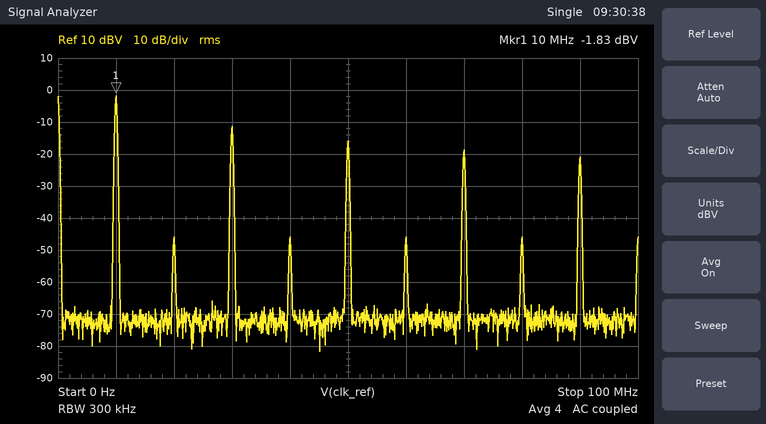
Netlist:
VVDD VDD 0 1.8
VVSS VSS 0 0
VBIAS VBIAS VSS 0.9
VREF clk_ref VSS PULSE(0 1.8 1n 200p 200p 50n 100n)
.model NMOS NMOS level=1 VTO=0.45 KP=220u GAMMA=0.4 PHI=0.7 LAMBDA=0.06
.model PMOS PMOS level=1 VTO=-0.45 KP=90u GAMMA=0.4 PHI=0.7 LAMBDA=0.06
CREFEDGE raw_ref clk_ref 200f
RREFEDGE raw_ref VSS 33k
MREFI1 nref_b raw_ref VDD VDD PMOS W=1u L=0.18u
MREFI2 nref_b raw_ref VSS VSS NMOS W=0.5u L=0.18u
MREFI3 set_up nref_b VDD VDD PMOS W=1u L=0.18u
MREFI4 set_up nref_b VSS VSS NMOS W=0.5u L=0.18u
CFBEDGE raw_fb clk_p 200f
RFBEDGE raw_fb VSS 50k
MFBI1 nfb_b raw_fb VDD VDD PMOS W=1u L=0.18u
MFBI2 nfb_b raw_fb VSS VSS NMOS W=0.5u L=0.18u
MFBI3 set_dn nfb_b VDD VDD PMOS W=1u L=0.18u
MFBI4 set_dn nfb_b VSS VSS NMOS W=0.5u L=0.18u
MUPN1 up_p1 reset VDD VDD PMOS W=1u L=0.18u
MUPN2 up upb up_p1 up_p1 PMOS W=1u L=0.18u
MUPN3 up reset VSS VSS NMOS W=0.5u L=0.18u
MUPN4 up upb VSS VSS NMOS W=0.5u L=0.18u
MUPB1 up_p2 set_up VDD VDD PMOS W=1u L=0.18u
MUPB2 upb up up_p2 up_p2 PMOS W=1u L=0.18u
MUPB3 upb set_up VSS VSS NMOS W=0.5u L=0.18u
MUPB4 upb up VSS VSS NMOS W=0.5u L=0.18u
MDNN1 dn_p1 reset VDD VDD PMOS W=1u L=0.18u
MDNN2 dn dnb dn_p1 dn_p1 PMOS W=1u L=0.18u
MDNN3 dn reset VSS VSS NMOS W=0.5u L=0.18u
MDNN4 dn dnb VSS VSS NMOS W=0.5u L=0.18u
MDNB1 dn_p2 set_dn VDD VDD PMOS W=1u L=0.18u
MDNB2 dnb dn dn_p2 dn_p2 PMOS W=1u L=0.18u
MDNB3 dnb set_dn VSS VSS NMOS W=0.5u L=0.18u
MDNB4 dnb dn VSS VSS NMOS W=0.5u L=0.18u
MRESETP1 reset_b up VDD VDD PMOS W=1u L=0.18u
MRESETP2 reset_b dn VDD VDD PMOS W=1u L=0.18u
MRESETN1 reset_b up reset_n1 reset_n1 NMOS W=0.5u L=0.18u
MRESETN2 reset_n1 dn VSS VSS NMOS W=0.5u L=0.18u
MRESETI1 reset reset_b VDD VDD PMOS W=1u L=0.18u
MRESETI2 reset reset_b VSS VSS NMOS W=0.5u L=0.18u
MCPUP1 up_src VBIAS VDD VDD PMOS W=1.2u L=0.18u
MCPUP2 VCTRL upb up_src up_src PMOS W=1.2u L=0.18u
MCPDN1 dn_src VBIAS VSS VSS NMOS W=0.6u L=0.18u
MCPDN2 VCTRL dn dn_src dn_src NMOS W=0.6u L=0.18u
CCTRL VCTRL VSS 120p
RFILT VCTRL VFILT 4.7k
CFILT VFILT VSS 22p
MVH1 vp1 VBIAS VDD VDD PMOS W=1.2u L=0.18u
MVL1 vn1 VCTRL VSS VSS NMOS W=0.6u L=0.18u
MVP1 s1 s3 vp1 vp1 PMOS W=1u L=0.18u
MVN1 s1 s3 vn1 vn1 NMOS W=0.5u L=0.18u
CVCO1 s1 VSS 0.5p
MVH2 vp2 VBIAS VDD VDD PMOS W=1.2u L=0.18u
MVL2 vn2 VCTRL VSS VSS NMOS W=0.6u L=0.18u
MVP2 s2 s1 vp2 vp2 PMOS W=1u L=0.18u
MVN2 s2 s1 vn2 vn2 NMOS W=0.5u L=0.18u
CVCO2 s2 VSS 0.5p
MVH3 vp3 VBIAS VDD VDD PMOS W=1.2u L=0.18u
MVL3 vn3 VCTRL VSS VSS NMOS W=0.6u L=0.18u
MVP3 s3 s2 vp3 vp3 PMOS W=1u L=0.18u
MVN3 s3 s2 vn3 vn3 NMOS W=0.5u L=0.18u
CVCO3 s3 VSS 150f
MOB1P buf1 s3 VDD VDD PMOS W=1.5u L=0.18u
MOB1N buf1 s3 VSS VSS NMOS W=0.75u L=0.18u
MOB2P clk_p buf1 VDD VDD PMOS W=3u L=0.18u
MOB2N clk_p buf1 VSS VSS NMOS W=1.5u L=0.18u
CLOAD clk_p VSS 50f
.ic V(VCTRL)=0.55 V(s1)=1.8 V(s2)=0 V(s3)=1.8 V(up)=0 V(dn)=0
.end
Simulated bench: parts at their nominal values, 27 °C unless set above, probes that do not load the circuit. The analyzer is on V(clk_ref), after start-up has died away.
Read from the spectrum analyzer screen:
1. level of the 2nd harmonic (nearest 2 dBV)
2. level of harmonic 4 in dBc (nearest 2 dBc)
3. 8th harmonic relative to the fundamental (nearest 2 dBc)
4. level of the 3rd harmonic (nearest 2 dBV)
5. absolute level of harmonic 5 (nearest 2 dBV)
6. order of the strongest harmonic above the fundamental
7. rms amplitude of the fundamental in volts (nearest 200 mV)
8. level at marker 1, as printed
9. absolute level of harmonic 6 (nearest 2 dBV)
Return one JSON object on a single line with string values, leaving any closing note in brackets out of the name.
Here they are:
{"level of the 2nd harmonic": "-46 dBV", "level of harmonic 4 in dBc": "-44 dBc", "8th harmonic relative to the fundamental": "-44 dBc", "level of the 3rd harmonic": "-12 dBV", "absolute level of harmonic 5": "-16 dBV", "order of the strongest harmonic above the fundamental": "3", "rms amplitude of the fundamental in volts": "800 mV", "level at marker 1, as printed": "-1.83 dBV", "absolute level of harmonic 6": "-46 dBV"}
